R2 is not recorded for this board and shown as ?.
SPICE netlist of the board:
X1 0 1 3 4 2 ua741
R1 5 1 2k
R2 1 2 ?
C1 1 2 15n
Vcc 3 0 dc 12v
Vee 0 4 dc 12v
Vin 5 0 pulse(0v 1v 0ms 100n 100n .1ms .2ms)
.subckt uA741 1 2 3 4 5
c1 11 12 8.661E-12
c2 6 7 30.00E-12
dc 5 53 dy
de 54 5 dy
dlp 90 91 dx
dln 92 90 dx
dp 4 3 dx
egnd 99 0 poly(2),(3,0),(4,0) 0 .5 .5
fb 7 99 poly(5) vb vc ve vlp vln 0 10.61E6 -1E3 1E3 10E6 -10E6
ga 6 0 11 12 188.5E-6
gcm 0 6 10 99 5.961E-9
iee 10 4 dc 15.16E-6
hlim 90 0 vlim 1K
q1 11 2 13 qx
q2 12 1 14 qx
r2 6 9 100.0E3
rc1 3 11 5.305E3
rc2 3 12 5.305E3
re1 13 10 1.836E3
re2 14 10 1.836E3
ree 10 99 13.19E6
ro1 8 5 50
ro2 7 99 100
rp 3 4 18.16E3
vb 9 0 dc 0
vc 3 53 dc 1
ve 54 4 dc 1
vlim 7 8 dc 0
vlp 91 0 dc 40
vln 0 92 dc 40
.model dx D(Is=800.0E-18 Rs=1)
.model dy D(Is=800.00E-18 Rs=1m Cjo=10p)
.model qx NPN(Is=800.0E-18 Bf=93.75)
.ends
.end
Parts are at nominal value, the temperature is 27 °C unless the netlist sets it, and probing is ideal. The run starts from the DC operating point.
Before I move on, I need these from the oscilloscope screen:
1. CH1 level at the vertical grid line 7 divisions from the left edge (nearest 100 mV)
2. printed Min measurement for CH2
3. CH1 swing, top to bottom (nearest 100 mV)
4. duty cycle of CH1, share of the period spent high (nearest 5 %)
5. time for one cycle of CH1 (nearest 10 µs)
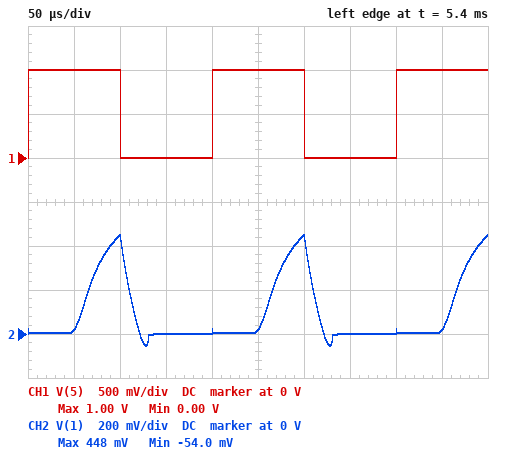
0 V
-54.0 mV
1.0 V
50 %
200 µs
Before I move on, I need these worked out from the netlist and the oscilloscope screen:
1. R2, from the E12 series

56 kΩ
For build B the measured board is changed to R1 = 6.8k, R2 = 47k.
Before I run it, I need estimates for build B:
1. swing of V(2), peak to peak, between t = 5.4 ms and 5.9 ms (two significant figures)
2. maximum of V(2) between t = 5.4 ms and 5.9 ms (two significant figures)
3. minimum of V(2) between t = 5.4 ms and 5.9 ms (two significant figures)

500 mV
-3.2 V
-3.7 V
